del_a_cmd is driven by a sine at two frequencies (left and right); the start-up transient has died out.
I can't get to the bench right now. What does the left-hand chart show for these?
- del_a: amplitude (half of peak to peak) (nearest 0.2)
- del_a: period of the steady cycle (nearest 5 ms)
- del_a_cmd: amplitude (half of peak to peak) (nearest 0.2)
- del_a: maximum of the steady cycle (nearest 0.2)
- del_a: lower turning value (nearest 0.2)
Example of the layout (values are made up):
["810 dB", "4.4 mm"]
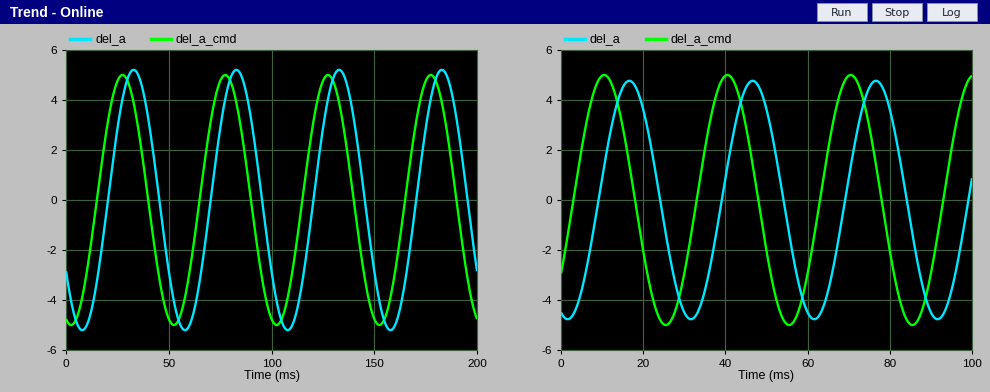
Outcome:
["5.2", "50 ms", "5.0", "5.2", "-5.2"]
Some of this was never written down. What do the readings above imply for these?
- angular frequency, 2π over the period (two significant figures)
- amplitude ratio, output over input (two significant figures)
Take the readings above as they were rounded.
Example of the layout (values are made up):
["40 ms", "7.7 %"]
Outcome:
["0.13 rad/ms", "1.0"]
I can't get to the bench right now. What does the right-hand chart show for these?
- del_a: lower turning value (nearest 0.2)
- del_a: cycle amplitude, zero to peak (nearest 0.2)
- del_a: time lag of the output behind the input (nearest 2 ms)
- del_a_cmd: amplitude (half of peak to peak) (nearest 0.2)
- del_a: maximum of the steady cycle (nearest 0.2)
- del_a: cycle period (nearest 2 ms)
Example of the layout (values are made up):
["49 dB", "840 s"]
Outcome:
["-4.8", "4.8", "6 ms", "5.0", "4.8", "30 ms"]
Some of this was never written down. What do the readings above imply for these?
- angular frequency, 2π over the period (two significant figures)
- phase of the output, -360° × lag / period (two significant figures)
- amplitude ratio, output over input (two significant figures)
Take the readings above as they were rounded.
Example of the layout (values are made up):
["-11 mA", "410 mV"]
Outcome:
["0.21 rad/ms", "-72°", "0.96"]
